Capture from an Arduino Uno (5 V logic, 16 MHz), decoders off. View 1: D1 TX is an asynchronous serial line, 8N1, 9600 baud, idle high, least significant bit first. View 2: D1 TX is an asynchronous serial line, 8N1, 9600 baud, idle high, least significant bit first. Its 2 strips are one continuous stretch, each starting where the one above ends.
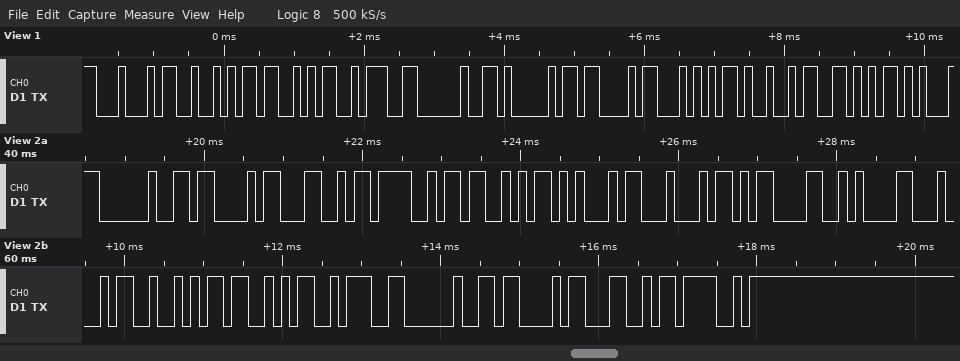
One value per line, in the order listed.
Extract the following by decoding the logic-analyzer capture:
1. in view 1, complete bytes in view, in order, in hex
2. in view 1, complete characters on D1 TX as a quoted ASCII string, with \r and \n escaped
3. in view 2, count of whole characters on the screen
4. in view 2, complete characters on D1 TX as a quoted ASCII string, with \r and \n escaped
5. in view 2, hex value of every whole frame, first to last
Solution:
0x44 0x52 0x53 0x3A 0x20 0x41 0x43 0x54 0x49 0x56
"DRS: ACTIV"
17
" CLOSED\r\nDRS: CLO"
20 43 4C 4F 53 45 44 0D 0A 44 52 53 3A 20 43 4C 4F
